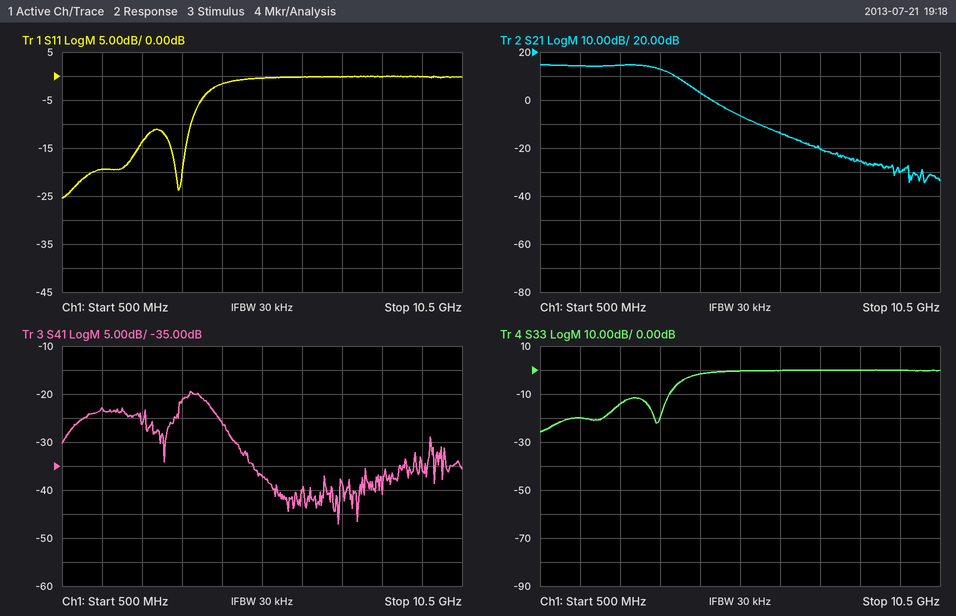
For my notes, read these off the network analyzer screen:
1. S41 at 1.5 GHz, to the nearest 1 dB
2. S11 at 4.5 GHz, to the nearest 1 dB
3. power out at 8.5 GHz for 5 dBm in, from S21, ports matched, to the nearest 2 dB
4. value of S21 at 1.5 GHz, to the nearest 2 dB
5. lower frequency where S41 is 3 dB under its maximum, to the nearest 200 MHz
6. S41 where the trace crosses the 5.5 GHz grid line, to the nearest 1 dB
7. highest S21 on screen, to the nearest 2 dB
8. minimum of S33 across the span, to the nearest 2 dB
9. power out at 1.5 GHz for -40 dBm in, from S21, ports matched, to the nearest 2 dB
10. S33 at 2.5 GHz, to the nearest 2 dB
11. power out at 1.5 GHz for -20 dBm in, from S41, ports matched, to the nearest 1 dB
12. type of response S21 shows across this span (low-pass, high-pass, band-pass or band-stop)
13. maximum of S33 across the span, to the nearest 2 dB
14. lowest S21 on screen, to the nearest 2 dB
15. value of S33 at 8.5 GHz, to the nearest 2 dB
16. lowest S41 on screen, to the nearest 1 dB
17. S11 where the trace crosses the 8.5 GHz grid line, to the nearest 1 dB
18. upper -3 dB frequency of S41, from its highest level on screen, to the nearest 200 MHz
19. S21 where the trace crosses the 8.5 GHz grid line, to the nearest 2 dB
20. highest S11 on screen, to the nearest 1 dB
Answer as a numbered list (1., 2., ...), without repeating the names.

1. -23 dB
2. -2 dB
3. -20 dBm
4. 14 dB
5. 3.4 GHz
6. -37 dB
7. 14 dB
8. -26 dB
9. -26 dBm
10. -14 dB
11. -43 dBm
12. low-pass
13. 0 dB
14. -34 dB
15. 0 dB
16. -47 dB
17. 0 dB
18. 4.2 GHz
19. -26 dB
20. 0 dB
